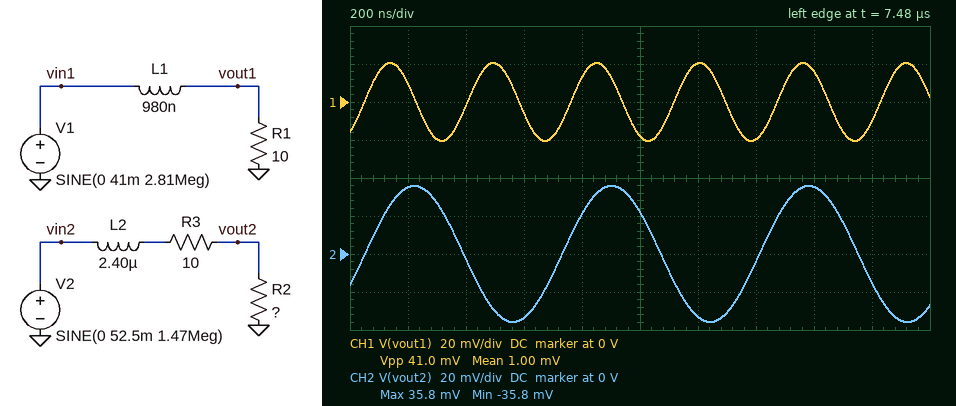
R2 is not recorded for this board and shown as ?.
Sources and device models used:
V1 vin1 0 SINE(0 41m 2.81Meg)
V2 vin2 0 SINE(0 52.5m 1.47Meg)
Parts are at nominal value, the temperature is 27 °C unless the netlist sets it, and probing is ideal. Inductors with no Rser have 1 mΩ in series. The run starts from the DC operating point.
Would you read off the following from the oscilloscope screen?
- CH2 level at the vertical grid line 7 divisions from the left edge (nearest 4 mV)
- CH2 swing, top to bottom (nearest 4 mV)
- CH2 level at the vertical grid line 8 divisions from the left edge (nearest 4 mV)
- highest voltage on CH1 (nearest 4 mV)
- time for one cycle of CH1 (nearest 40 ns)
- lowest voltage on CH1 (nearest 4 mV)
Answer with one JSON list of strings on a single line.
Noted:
["-4 mV", "72 mV", "36 mV", "20 mV", "360 ns", "-20 mV"]
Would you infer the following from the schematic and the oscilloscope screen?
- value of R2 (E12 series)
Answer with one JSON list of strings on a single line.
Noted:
["33 Ω"]
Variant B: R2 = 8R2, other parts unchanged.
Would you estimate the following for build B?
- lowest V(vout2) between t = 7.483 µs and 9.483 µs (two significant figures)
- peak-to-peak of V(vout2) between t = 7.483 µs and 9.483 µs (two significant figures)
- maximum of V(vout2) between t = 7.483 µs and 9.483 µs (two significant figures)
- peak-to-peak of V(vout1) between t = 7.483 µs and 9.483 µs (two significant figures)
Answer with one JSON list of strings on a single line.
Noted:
["-15 mV", "30 mV", "15 mV", "41 mV"]
